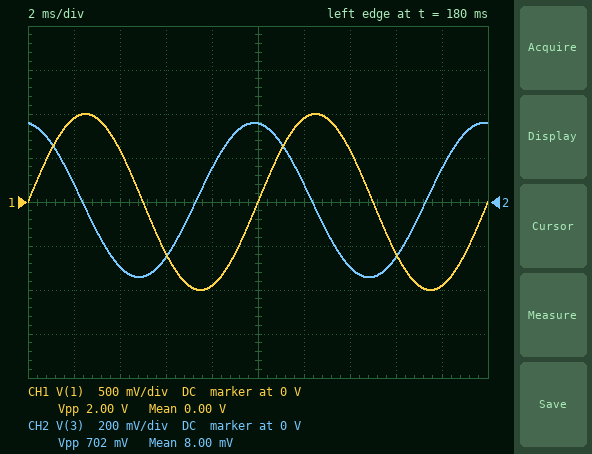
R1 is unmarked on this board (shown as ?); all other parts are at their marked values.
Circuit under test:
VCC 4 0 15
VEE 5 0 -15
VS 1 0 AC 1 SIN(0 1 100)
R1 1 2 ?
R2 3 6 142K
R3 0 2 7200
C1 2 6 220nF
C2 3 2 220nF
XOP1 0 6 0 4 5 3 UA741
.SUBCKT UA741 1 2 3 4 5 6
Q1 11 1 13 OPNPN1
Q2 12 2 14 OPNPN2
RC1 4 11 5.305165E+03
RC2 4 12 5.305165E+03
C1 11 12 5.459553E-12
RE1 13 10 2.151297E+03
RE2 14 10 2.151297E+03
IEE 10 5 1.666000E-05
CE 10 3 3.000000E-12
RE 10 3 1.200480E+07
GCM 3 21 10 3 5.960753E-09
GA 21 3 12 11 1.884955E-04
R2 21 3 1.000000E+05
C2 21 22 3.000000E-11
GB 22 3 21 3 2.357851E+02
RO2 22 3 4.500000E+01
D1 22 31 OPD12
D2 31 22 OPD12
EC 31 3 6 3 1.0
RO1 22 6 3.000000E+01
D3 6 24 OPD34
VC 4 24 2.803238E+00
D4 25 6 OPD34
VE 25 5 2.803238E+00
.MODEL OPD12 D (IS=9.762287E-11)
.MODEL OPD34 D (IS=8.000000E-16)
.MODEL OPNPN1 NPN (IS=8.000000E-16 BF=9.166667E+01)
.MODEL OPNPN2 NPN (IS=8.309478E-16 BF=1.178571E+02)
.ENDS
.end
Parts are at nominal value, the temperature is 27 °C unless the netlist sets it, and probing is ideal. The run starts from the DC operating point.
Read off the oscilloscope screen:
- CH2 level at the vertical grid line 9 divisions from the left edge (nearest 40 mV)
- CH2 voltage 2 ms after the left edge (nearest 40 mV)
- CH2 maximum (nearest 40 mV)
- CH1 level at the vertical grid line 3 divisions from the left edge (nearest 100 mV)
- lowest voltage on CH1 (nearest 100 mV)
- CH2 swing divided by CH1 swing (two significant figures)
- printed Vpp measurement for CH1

160 mV
80 mV
360 mV
-600 mV
-1.0 V
0.35
2.00 V
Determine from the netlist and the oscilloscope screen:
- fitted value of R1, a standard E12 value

22 kΩ
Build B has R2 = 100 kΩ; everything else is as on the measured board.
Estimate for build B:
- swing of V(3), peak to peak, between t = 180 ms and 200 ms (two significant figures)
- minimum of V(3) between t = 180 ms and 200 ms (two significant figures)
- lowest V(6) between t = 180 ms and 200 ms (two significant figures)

720 mV
-350 mV
-1.0 mV
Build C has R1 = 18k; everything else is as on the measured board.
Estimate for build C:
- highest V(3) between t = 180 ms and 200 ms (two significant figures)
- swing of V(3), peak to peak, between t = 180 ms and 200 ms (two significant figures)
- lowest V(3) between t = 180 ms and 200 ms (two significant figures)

440 mV
860 mV
-420 mV
